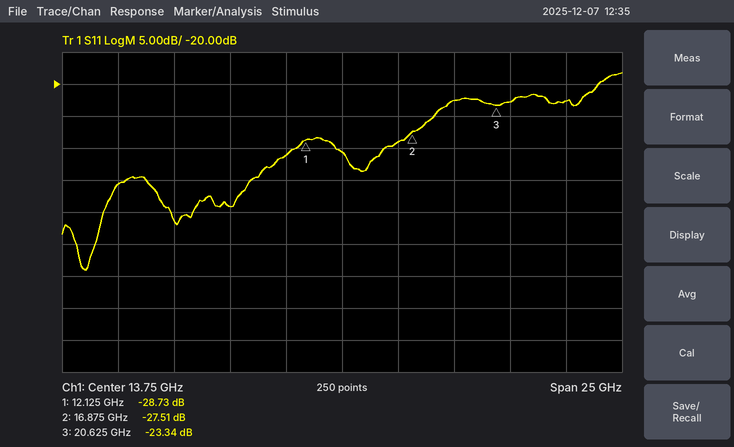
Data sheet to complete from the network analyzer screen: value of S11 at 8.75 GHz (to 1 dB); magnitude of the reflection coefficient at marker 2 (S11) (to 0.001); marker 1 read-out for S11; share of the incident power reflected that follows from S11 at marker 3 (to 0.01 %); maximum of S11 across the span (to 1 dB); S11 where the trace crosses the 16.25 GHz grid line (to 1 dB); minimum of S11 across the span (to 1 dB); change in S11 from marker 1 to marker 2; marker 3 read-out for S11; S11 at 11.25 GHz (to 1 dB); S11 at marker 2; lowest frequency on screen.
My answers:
-39 dB
0.042
-28.73 dB
0.46 %
-18 dB
-29 dB
-49 dB
1.22 dB
-23.34 dB
-31 dB
-27.51 dB
1.25 GHz
